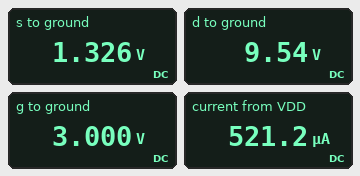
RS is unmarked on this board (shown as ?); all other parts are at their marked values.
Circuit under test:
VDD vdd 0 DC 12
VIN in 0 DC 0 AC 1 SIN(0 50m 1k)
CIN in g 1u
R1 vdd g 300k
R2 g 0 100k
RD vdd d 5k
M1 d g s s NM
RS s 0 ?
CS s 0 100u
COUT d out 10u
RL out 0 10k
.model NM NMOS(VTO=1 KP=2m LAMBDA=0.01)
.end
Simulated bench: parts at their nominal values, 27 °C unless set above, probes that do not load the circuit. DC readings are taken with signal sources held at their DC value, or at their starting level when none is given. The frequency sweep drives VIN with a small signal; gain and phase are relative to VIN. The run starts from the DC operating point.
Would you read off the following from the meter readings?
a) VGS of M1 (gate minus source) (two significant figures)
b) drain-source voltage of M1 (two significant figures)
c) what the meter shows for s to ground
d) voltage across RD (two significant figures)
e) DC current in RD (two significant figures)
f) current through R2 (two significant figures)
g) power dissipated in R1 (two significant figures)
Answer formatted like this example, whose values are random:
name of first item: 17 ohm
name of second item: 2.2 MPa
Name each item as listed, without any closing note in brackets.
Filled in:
VGS of M1 (gate minus source): 1.7 V
drain-source voltage of M1: 8.2 V
what the meter shows for s to ground: 1.326 V
voltage across RD: 2.5 V
DC current in RD: 490 µA
current through R2: 30 µA
power dissipated in R1: 270 µW
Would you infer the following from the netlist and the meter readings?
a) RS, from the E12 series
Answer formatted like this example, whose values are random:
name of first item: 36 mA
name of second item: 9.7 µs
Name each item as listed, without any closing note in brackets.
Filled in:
RS, from the E12 series: 2.7 kΩ
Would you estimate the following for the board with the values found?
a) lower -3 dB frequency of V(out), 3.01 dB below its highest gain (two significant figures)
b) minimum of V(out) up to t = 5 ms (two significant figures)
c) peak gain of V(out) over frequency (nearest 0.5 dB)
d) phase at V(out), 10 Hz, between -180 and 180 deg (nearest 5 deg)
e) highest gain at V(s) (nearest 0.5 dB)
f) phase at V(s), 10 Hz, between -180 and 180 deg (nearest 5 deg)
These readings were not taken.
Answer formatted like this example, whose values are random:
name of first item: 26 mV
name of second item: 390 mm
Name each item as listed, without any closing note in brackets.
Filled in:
lower -3 dB frequency of V(out), 3.01 dB below its highest gain: 4.1 Hz
minimum of V(out) up to t = 5 ms: -250 mV
peak gain of V(out) over frequency: 13.5 dB
phase at V(out), 10 Hz, between -180 and 180 deg: -150 deg
highest gain at V(s): -7.0 dB
phase at V(s), 10 Hz, between -180 and 180 deg: -60 deg
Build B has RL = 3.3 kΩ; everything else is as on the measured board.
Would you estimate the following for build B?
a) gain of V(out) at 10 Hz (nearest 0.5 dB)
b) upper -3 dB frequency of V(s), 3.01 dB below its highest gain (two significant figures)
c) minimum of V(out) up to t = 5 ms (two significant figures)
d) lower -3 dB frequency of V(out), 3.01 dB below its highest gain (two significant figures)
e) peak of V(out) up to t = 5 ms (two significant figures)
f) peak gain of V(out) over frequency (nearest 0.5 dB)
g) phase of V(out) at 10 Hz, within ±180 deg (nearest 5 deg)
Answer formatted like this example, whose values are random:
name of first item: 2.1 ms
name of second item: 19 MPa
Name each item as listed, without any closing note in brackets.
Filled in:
gain of V(out) at 10 Hz: 8.5 dB
upper -3 dB frequency of V(s), 3.01 dB below its highest gain: 6.1 Hz
minimum of V(out) up to t = 5 ms: -150 mV
lower -3 dB frequency of V(out), 3.01 dB below its highest gain: 4.5 Hz
peak of V(out) up to t = 5 ms: 140 mV
peak gain of V(out) over frequency: 9.0 dB
phase of V(out) at 10 Hz, within ±180 deg: -145 deg
